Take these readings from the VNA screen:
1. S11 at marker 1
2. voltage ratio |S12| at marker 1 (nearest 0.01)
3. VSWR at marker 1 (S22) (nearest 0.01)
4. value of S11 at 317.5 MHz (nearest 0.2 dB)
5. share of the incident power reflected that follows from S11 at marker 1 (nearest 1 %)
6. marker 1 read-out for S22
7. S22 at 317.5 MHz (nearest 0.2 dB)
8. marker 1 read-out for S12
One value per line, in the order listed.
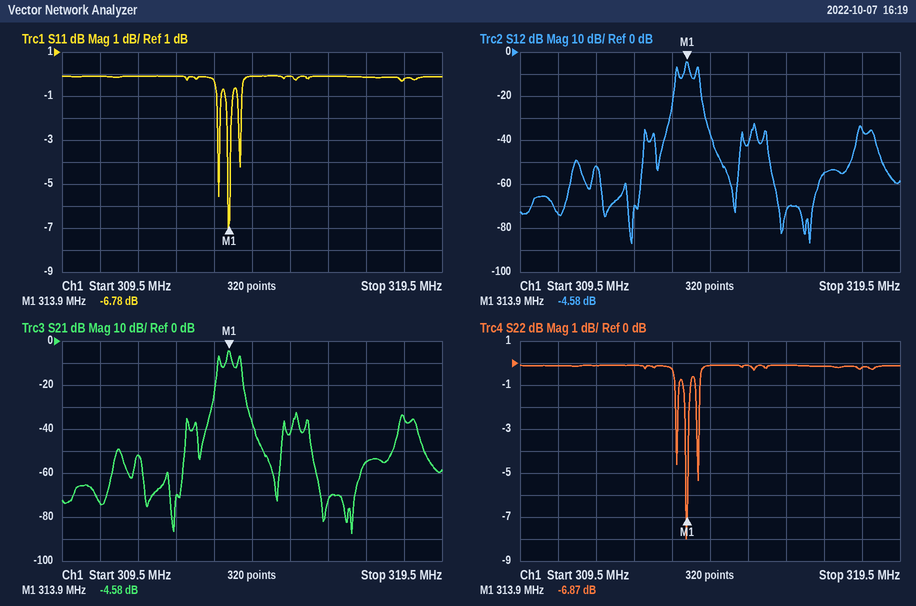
-6.78 dB
0.59
2.66
-0.2 dB
21 %
-6.87 dB
-0.2 dB
-4.58 dB
